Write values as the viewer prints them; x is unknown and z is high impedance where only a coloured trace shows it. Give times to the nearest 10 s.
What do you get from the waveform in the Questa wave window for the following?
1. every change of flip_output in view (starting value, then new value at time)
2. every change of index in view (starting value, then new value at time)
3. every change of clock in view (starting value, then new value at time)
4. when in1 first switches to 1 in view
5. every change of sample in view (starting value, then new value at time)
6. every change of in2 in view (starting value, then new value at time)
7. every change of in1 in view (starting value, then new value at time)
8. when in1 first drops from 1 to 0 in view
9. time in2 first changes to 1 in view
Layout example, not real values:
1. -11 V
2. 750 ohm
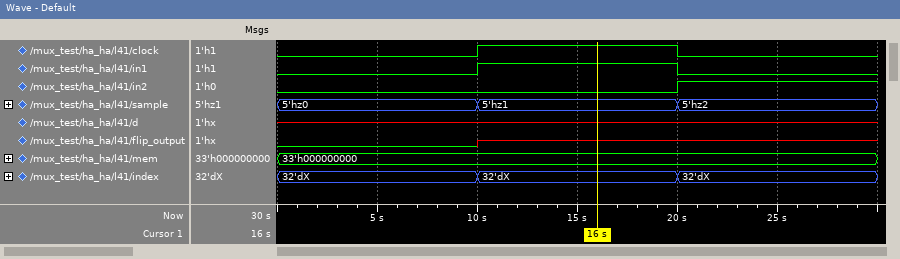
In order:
1. 0, x at 10 s
2. 32'dX, 32'dX at 10 s, 32'dX at 20 s
3. 0, 1 at 10 s, 0 at 20 s
4. 10 s
5. 5'hz0, 5'hz1 at 10 s, 5'hz2 at 20 s
6. 0, 1 at 20 s
7. 0, 1 at 10 s, 0 at 20 s
8. 20 s
9. 20 s
